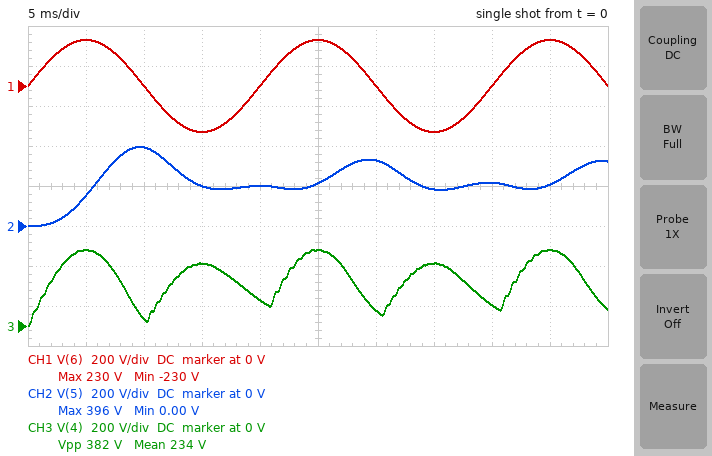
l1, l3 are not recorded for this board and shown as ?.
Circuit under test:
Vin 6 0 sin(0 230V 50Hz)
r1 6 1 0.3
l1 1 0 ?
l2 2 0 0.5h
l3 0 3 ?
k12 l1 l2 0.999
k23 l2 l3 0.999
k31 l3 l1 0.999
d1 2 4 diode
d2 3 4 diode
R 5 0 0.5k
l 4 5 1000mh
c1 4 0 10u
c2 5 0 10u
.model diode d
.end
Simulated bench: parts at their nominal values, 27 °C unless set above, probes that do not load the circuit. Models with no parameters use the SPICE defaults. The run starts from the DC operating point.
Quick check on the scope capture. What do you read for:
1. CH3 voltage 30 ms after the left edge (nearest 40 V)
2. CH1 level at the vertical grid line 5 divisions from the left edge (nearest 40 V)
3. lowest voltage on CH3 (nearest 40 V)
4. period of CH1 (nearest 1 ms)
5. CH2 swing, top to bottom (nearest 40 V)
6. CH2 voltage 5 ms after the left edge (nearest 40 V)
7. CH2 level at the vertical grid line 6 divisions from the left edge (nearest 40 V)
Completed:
80 V
240 V
0 V
20 ms
400 V
160 V
320 V
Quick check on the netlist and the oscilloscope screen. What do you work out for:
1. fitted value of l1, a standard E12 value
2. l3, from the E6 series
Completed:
180 mH
330 mH
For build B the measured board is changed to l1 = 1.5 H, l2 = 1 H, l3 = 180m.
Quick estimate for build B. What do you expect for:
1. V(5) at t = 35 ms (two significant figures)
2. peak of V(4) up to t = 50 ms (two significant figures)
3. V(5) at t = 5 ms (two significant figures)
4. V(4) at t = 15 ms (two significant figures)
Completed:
59 V
190 V
74 V
86 V
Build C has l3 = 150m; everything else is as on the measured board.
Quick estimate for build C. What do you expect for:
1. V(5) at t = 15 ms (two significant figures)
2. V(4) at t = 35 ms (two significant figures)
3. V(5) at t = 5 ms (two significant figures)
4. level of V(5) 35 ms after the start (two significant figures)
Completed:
160 V
210 V
150 V
140 V
